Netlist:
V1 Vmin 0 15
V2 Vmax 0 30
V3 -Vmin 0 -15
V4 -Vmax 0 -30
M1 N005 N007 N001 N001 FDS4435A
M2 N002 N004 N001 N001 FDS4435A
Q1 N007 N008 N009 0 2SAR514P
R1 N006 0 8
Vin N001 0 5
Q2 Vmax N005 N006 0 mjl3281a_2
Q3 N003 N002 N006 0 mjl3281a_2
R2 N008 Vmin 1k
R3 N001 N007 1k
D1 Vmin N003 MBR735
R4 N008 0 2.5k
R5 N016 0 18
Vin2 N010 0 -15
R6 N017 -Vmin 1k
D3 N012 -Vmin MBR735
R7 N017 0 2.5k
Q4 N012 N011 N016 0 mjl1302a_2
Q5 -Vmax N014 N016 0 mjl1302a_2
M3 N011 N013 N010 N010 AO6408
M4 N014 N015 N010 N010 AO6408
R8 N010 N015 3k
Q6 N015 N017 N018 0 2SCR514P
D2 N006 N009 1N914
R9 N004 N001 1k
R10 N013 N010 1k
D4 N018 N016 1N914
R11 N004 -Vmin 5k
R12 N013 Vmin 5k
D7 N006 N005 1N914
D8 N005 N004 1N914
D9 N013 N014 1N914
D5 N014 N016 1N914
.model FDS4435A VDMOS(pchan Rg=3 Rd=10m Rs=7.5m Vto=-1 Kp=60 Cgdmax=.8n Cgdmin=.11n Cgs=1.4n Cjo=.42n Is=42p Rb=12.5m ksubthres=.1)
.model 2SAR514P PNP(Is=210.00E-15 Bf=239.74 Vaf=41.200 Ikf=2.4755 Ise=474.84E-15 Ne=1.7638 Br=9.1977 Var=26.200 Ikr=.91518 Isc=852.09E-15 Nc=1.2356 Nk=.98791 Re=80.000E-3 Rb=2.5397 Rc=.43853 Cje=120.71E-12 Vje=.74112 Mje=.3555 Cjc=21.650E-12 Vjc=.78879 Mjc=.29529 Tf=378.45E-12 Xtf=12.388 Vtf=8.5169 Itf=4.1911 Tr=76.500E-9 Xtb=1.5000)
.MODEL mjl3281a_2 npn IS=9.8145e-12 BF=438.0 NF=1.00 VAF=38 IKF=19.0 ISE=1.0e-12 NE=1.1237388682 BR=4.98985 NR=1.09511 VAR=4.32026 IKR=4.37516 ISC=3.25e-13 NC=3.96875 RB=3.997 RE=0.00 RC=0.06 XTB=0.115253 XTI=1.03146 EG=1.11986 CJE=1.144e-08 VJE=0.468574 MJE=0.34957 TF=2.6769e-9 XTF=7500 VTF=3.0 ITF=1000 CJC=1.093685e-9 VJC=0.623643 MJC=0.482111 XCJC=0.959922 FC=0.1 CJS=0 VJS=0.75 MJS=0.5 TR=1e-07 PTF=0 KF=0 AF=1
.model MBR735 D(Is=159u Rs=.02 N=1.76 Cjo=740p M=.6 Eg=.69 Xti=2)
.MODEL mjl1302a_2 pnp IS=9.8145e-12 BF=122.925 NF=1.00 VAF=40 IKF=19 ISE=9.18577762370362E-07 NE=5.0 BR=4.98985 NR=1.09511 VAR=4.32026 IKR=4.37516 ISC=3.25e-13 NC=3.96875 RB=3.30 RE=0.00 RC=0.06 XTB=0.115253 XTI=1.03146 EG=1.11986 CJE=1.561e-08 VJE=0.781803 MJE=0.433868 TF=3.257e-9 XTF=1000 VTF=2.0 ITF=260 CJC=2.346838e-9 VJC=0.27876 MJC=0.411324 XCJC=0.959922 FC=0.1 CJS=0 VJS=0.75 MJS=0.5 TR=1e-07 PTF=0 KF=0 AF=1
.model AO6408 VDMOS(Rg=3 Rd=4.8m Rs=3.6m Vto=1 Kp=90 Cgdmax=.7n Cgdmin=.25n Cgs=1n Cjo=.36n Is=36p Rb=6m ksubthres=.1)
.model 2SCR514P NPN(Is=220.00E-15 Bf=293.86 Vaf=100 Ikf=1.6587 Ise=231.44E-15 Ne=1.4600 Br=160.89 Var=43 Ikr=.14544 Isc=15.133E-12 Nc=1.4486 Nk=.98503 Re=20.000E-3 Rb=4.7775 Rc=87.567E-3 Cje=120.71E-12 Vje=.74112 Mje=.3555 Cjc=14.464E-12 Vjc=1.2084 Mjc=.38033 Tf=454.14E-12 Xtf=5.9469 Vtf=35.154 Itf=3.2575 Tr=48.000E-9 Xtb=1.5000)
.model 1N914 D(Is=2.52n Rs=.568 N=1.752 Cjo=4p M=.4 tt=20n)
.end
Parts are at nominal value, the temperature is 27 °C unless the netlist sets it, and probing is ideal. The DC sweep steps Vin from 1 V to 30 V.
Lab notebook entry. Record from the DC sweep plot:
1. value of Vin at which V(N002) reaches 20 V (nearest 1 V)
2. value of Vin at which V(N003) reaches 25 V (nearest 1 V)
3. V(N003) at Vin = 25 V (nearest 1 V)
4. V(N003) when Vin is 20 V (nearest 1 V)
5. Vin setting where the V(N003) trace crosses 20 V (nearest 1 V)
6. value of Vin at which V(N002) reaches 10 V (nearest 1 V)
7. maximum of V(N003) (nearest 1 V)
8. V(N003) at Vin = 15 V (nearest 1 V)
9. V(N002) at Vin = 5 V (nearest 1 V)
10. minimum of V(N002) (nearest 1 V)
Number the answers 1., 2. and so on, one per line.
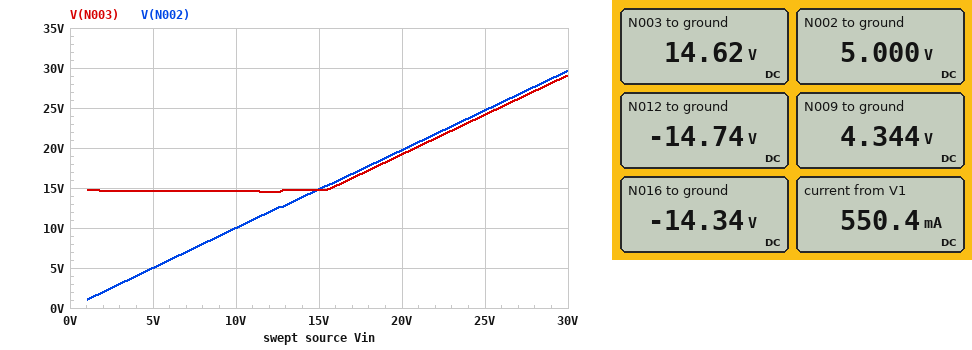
1. 20 V
2. 26 V
3. 24 V
4. 19 V
5. 21 V
6. 10 V
7. 29 V
8. 15 V
9. 5 V
10. 1 V
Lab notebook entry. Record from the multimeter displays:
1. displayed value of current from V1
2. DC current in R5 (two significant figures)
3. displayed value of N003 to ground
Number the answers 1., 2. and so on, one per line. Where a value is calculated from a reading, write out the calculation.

1. 550.4 mA
2. (0 V - (-14.34 V)) / 18 Ω = 800 mA
3. 14.62 V
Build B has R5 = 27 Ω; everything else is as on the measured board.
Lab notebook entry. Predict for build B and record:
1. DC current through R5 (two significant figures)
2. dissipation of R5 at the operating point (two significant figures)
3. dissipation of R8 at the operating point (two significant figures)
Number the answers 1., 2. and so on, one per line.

1. 530 mA
2. 7.6 W
3. 540 µW
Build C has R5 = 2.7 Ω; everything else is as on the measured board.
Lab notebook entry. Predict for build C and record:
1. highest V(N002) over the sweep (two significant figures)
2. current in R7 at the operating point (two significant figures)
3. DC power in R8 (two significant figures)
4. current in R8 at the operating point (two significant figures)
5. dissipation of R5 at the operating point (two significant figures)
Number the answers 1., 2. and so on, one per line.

1. 30 V
2. 5.1 mA
3. 720 µW
4. 490 µA
5. 74 W
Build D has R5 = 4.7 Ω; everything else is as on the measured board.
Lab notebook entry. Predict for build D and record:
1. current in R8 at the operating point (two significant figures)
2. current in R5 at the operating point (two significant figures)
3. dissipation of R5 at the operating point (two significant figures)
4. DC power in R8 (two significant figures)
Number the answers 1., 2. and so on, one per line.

1. 460 µA
2. 3.0 A
3. 43 W
4. 640 µW
